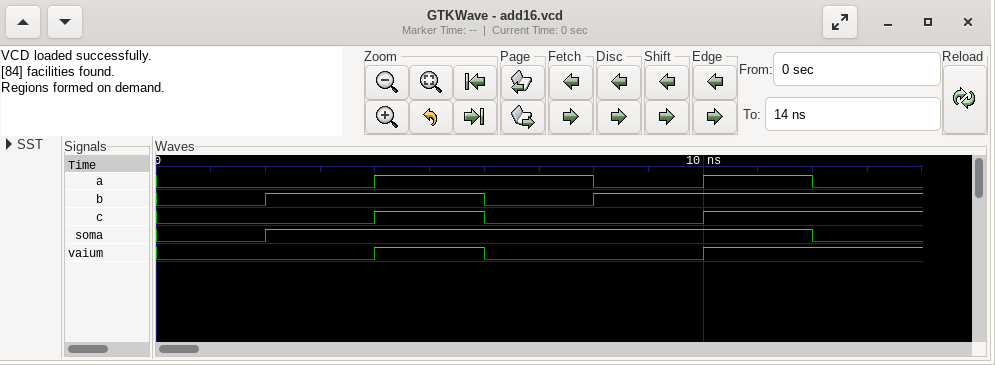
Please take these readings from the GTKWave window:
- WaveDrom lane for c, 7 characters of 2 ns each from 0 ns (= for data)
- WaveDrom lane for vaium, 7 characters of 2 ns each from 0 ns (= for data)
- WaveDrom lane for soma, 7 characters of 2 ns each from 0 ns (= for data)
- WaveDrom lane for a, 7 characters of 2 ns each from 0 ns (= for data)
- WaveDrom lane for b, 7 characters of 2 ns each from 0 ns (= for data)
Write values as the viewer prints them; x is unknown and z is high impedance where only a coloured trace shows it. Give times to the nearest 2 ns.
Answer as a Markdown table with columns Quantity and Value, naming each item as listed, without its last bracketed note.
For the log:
| Quantity | Value |
|---|---|
| WaveDrom lane for c, 7 characters of 2 ns each from 0 ns | {name: 'c', wave: '0.10.1.'} |
| WaveDrom lane for vaium, 7 characters of 2 ns each from 0 ns | {name: 'vaium', wave: '0.10.1.'} |
| WaveDrom lane for soma, 7 characters of 2 ns each from 0 ns | {name: 'soma', wave: '01....0'} |
| WaveDrom lane for a, 7 characters of 2 ns each from 0 ns | {name: 'a', wave: '0.1.010'} |
| WaveDrom lane for b, 7 characters of 2 ns each from 0 ns | {name: 'b', wave: '01.01..'} |
